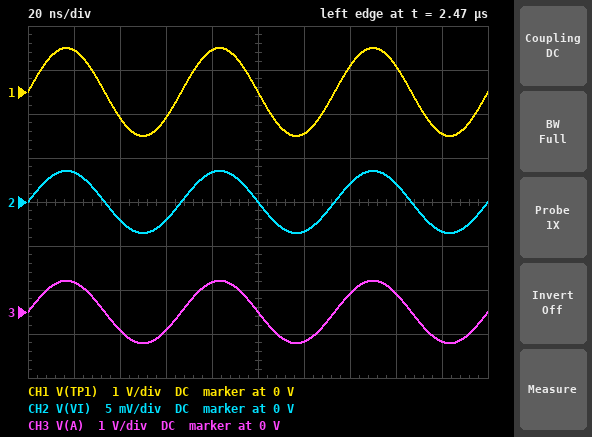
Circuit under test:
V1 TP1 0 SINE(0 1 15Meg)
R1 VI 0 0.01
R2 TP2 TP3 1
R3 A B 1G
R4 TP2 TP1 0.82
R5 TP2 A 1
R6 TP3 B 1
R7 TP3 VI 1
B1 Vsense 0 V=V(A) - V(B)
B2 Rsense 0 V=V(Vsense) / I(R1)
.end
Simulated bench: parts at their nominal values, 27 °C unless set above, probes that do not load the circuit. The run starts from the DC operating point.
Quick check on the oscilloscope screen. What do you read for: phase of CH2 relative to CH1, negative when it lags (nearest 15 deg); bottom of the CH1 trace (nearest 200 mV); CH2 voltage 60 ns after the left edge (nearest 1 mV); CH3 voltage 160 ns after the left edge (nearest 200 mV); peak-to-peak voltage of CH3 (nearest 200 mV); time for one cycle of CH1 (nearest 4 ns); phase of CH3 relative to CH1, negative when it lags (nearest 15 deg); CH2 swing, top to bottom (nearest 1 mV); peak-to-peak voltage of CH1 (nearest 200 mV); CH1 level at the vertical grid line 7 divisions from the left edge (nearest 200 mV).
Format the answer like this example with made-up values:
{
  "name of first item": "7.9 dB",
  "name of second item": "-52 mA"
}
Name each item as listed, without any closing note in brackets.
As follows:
{
  "phase of CH2 relative to CH1, negative when it lags": "0 deg",
  "bottom of the CH1 trace": "-1.0 V",
  "CH2 voltage 60 ns after the left edge": "-2 mV",
  "CH3 voltage 160 ns after the left edge": "400 mV",
  "peak-to-peak voltage of CH3": "1.4 V",
  "time for one cycle of CH1": "68 ns",
  "phase of CH3 relative to CH1, negative when it lags": "0 deg",
  "CH2 swing, top to bottom": "7 mV",
  "peak-to-peak voltage of CH1": "2.0 V",
  "CH1 level at the vertical grid line 7 divisions from the left edge": "600 mV"
}
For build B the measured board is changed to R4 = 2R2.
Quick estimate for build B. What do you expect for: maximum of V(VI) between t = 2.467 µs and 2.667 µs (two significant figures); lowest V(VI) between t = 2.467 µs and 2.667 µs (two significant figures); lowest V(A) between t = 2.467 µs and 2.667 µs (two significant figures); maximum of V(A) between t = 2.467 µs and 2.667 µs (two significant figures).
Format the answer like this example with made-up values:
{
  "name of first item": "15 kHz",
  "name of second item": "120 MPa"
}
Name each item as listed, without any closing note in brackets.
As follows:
{
  "maximum of V(VI) between t = 2.467 µs and 2.667 µs": "2.4 mV",
  "lowest V(VI) between t = 2.467 µs and 2.667 µs": "-2.4 mV",
  "lowest V(A) between t = 2.467 µs and 2.667 µs": "-480 mV",
  "maximum of V(A) between t = 2.467 µs and 2.667 µs": "480 mV"
}
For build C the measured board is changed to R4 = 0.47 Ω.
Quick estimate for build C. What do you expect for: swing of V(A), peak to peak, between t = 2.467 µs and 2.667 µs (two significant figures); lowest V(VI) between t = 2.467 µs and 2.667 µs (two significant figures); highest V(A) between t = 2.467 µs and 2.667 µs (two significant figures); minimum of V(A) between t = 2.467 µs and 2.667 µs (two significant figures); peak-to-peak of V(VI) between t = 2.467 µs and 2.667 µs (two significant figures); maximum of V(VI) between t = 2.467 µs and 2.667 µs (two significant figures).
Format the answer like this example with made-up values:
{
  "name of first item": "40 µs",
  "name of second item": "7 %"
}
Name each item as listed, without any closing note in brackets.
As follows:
{
  "swing of V(A), peak to peak, between t = 2.467 µs and 2.667 µs": "1.6 V",
  "lowest V(VI) between t = 2.467 µs and 2.667 µs": "-4.0 mV",
  "highest V(A) between t = 2.467 µs and 2.667 µs": "810 mV",
  "minimum of V(A) between t = 2.467 µs and 2.667 µs": "-810 mV",
  "peak-to-peak of V(VI) between t = 2.467 µs and 2.667 µs": "8.1 mV",
  "maximum of V(VI) between t = 2.467 µs and 2.667 µs": "4.0 mV"
}
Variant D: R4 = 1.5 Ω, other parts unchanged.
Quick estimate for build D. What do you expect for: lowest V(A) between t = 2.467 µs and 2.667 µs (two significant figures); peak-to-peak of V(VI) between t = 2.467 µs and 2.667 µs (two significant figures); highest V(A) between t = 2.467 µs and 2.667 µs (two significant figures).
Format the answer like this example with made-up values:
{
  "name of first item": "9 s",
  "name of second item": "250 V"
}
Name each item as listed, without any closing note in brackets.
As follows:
{
  "lowest V(A) between t = 2.467 µs and 2.667 µs": "-570 mV",
  "peak-to-peak of V(VI) between t = 2.467 µs and 2.667 µs": "5.7 mV",
  "highest V(A) between t = 2.467 µs and 2.667 µs": "570 mV"
}
